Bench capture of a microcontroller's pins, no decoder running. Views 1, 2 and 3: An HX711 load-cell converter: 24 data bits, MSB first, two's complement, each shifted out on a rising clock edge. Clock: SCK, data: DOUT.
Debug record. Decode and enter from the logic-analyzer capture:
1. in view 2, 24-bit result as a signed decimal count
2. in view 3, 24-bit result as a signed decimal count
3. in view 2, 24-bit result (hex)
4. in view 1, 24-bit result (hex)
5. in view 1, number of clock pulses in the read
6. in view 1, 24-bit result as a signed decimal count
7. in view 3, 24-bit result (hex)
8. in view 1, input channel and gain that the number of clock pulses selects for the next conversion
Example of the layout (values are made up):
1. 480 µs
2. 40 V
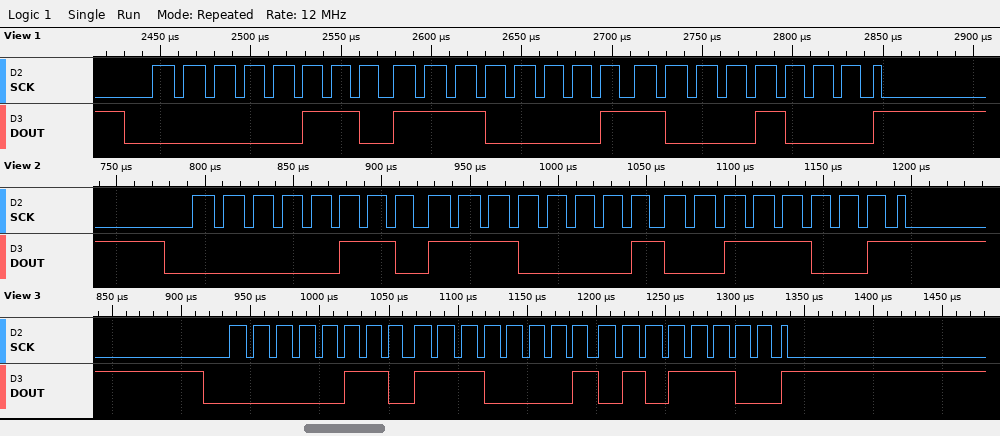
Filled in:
1. 450873
2. 450908
3. 0x06E139
4. 0x06E188
5. 25
6. 450952
7. 0x06E15C
8. channel A, gain 128
